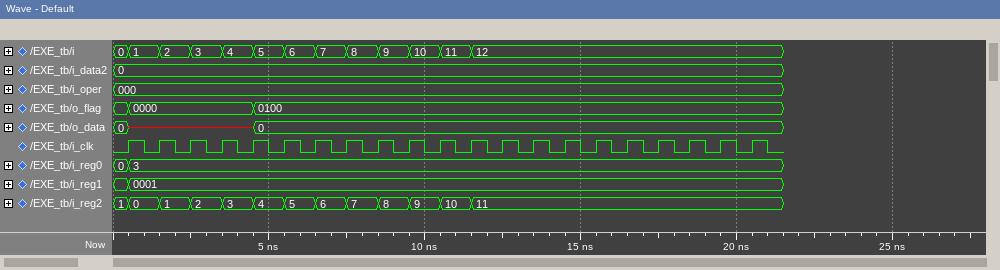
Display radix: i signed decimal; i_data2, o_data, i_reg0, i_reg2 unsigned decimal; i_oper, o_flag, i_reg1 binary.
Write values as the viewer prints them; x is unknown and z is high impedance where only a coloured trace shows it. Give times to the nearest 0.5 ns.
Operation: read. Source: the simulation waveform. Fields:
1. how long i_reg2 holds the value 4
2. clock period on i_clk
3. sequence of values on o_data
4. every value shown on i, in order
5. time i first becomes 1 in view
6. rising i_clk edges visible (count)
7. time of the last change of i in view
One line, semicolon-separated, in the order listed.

1 ns; 1 ns; 0, x, 0; 0, 1, 2, 3, 4, 5, 6, 7, 8, 9, 10, 11, 12; 0.5 ns; 21; 11.5 ns
